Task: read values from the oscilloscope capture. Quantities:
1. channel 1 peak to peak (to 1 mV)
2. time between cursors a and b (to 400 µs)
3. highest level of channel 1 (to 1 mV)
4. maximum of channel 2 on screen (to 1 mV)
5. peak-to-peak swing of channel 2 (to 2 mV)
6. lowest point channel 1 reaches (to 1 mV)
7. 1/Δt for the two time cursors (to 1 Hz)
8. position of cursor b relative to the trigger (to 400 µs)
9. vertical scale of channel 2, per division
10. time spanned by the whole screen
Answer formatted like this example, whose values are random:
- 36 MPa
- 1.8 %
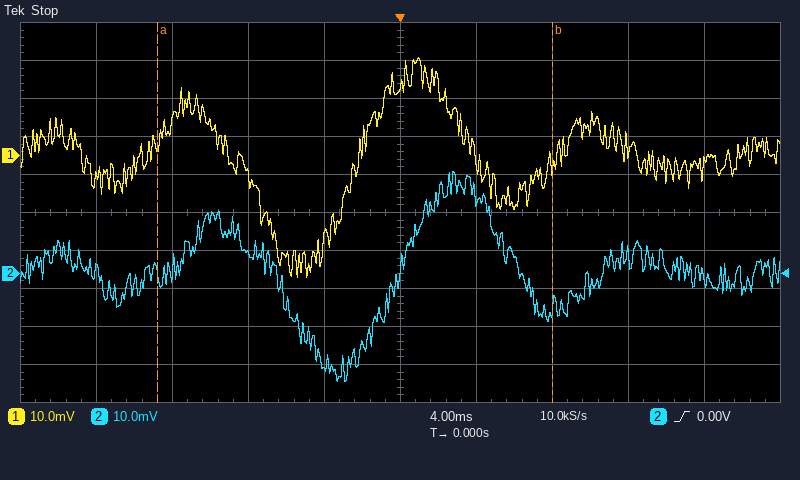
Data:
- 58 mV
- 20.8 ms
- 26 mV
- 27 mV
- 56 mV
- -32 mV
- 48 Hz
- +8.0 ms
- 10 mV
- 40 ms
